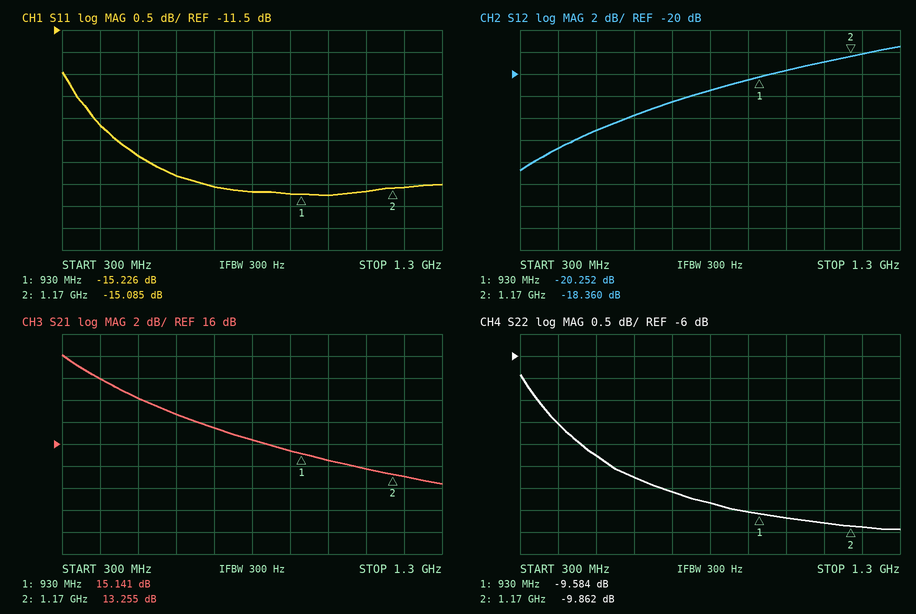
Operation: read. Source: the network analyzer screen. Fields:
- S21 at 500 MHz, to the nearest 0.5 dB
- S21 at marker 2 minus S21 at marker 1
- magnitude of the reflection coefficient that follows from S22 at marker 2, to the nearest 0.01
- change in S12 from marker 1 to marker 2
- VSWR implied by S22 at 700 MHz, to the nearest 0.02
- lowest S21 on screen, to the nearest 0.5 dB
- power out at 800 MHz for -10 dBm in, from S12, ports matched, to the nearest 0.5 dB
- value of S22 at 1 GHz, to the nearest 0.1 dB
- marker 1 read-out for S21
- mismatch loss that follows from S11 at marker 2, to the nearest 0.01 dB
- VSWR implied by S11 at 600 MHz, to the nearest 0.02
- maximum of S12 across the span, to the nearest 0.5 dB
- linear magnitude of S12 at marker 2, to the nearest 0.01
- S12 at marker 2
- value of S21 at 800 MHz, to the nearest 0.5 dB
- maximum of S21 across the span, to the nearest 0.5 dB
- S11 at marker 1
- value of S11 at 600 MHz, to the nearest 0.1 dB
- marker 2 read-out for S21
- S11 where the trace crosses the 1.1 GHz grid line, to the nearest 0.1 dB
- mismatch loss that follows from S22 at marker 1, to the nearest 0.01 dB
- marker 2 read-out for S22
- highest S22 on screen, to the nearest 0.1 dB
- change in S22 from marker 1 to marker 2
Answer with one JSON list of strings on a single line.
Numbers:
["20.0 dB", "-1.886 dB", "0.32", "1.892 dB", "2.08", "12.5 dB", "-31.5 dBm", "-9.7 dB", "15.141 dB", "0.14 dB", "1.44", "-17.5 dB", "0.12", "-18.360 dB", "16.5 dB", "24.0 dB", "-15.226 dB", "-14.8 dB", "13.255 dB", "-15.2 dB", "0.51 dB", "-9.862 dB", "-6.4 dB", "-0.278 dB"]
